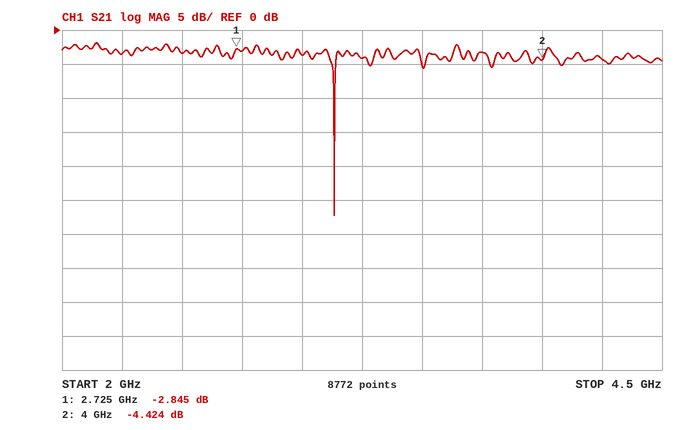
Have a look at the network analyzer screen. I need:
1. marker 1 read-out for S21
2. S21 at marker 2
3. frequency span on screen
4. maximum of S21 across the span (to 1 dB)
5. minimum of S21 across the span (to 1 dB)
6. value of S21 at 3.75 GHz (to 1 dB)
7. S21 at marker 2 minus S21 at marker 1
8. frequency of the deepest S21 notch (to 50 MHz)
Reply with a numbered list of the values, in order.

1. -2.845 dB
2. -4.424 dB
3. 2.5 GHz
4. -2 dB
5. -27 dB
6. -3 dB
7. -1.579 dB
8. 3.15 GHz
